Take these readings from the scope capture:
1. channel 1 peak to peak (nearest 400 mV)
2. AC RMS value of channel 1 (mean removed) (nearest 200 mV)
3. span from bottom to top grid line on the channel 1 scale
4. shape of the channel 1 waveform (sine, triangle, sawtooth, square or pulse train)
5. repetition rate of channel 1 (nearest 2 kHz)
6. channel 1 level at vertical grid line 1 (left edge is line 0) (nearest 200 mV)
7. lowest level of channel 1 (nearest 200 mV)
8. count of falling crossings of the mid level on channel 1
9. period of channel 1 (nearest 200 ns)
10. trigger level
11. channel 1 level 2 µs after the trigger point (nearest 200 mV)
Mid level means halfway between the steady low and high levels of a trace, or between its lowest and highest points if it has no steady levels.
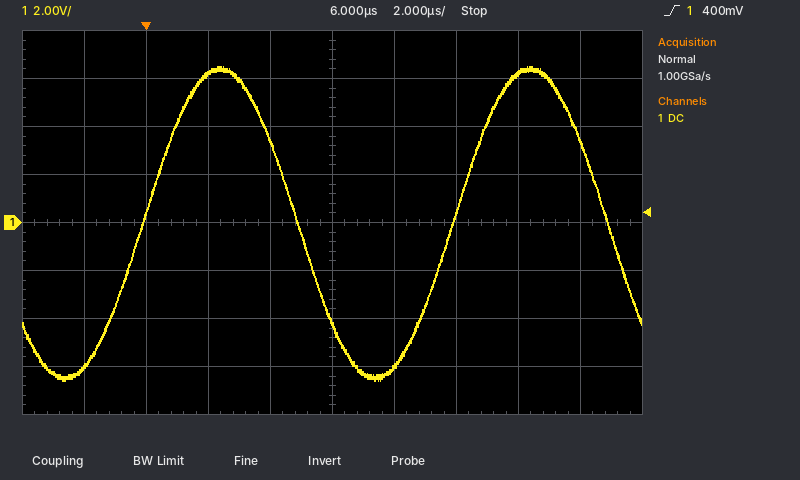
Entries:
13.2 V
4.6 V
16 V
sine
100 kHz
-6.0 V
-6.6 V
2
10.0 µs
400 mV
6.2 V
